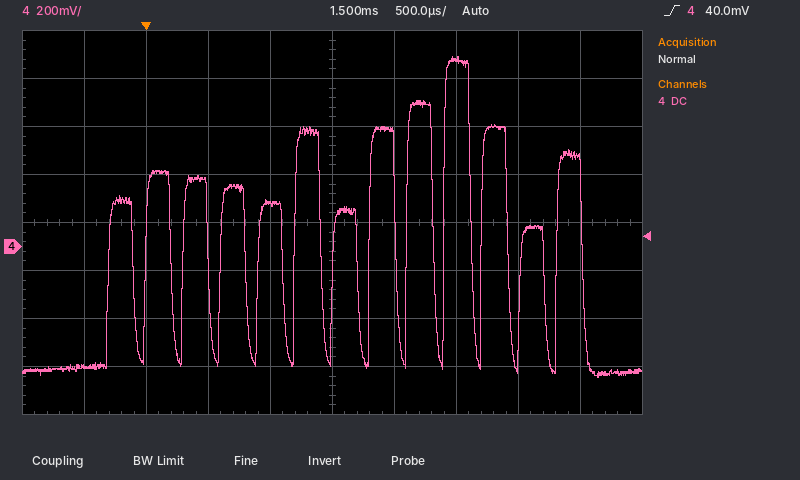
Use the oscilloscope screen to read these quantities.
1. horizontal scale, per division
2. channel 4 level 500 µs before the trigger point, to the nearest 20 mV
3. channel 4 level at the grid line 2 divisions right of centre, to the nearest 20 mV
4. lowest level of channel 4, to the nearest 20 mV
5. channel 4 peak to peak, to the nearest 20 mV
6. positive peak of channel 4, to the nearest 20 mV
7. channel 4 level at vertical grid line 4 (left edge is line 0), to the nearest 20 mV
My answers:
500 µs
-500 mV
780 mV
-540 mV
1.34 V
800 mV
180 mV
